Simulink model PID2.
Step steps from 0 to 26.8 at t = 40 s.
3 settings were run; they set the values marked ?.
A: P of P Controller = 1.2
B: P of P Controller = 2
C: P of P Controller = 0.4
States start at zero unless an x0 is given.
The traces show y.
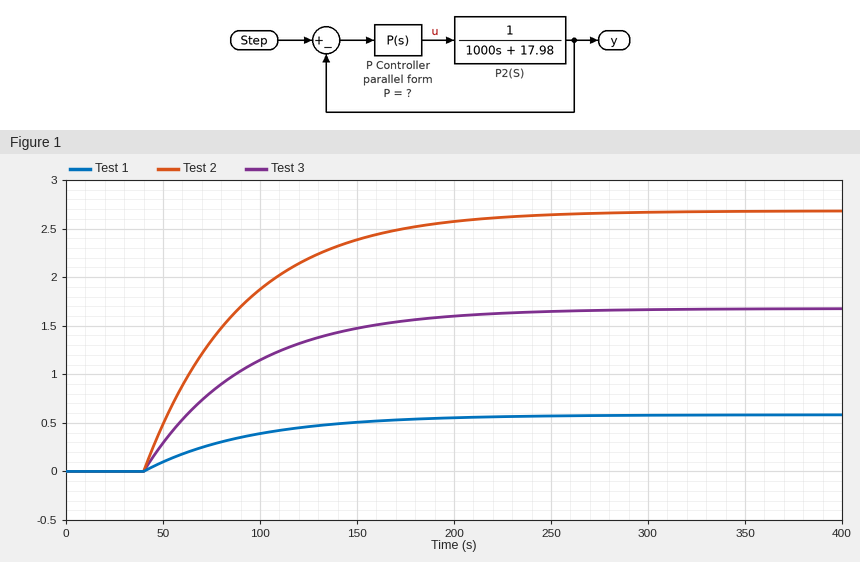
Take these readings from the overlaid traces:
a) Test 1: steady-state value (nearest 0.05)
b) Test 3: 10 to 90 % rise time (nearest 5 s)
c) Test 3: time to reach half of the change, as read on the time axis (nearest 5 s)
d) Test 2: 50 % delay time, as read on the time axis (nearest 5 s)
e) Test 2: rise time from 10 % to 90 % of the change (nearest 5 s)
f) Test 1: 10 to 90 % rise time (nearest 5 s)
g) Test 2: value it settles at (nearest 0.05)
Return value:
0.60
115 s
75 s
75 s
110 s
120 s
2.70
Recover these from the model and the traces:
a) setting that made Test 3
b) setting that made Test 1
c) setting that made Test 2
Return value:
A
C
B
